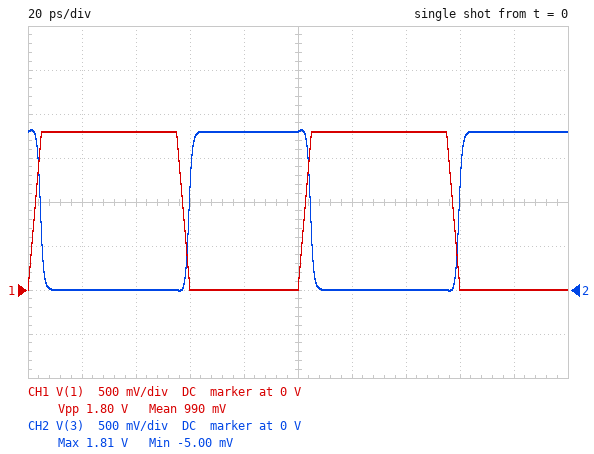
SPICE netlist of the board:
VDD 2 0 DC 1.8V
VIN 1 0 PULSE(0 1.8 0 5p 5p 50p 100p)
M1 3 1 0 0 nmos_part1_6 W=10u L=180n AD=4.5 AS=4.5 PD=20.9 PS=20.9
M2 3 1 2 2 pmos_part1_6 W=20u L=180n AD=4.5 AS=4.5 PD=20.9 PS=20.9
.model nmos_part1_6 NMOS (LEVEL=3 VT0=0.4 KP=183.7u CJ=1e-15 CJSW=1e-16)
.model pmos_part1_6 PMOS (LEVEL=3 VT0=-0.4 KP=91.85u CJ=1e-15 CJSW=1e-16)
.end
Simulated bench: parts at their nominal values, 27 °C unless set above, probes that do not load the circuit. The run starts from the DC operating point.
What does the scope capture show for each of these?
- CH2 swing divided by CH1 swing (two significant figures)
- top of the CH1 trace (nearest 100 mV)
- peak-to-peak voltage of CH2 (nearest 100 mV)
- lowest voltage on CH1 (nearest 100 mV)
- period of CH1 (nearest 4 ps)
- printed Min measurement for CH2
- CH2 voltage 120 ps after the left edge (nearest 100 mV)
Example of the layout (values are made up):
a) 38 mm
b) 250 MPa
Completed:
a) 1.0
b) 1.8 V
c) 1.8 V
d) 0 V
e) 100 ps
f) -5.00 mV
g) 0 V
